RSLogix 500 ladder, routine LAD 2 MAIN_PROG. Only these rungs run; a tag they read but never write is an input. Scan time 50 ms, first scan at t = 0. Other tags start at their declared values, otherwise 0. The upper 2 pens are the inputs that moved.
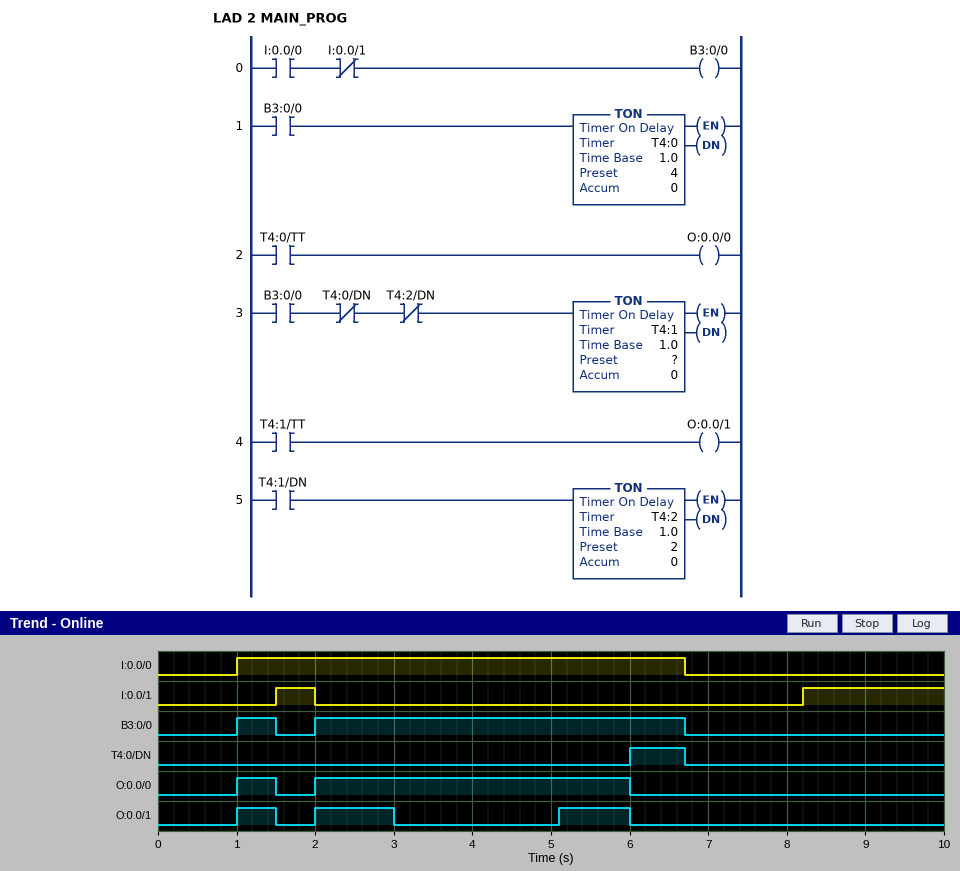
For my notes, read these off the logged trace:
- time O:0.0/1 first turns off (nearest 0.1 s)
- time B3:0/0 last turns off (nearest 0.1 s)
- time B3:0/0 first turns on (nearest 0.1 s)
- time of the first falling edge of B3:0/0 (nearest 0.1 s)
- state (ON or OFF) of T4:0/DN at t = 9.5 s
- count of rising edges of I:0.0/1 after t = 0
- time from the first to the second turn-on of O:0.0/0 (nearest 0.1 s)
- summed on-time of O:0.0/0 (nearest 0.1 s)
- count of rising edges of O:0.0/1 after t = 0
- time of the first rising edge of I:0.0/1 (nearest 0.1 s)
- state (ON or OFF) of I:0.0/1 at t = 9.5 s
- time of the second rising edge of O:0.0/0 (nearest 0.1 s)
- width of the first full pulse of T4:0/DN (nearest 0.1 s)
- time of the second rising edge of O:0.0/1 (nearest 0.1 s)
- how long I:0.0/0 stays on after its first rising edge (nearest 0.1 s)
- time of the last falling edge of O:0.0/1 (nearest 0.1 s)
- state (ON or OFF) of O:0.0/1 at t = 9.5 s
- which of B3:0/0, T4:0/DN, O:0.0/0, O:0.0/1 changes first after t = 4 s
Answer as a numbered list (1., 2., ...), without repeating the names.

1. 1.5 s
2. 6.7 s
3. 1.0 s
4. 1.5 s
5. OFF
6. 2
7. 1.0 s
8. 4.5 s
9. 3
10. 1.5 s
11. ON
12. 2.0 s
13. 0.7 s
14. 2.0 s
15. 5.7 s
16. 6.0 s
17. OFF
18. O:0.0/1
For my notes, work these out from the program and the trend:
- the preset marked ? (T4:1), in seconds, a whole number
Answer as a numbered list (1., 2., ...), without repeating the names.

1. 1 s
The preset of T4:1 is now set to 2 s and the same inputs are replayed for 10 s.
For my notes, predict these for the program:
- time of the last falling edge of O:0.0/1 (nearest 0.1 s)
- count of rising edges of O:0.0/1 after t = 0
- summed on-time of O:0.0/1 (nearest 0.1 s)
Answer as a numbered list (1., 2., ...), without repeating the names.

1. 4.0 s
2. 2
3. 2.5 s
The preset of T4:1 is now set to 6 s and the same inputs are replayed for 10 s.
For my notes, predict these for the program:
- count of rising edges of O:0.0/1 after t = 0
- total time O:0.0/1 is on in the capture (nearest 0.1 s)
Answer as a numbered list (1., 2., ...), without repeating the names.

1. 2
2. 4.5 s
